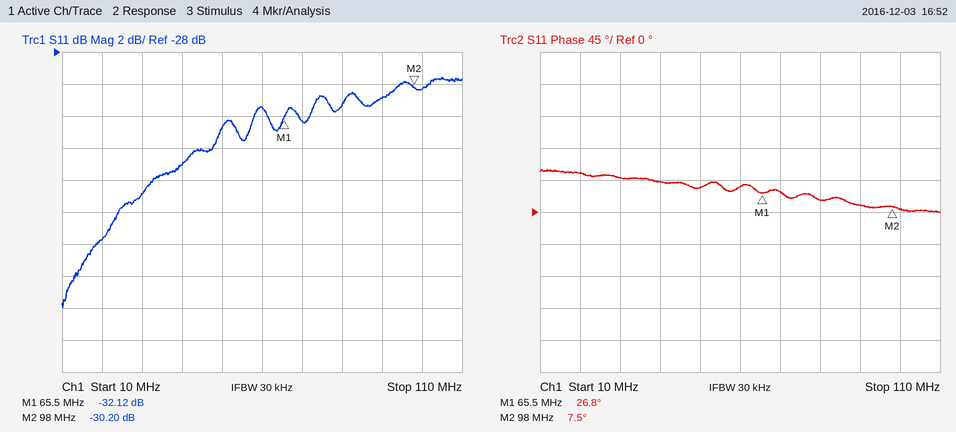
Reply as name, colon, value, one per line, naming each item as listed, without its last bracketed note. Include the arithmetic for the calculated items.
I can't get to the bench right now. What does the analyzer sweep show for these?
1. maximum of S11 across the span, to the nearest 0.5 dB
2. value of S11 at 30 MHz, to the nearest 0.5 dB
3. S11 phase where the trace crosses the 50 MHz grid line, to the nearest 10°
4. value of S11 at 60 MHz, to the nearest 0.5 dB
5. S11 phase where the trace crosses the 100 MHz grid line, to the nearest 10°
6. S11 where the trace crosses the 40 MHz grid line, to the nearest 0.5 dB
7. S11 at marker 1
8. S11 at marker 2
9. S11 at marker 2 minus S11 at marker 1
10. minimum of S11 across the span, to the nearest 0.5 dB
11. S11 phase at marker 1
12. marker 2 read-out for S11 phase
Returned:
maximum of S11 across the span, to the nearest 0.5 dB: -29.5 dB
value of S11 at 30 MHz, to the nearest 0.5 dB: -37.0 dB
S11 phase where the trace crosses the 50 MHz grid line, to the nearest 10°: 30°
value of S11 at 60 MHz, to the nearest 0.5 dB: -31.5 dB
S11 phase where the trace crosses the 100 MHz grid line, to the nearest 10°: 0°
S11 where the trace crosses the 40 MHz grid line, to the nearest 0.5 dB: -35.0 dB
S11 at marker 1: -32.12 dB
S11 at marker 2: -30.20 dB
S11 at marker 2 minus S11 at marker 1: -30.2 − (-32.12) = 1.92 dB
minimum of S11 across the span, to the nearest 0.5 dB: -44.0 dB
S11 phase at marker 1: 26.8°
marker 2 read-out for S11 phase: 7.5°
